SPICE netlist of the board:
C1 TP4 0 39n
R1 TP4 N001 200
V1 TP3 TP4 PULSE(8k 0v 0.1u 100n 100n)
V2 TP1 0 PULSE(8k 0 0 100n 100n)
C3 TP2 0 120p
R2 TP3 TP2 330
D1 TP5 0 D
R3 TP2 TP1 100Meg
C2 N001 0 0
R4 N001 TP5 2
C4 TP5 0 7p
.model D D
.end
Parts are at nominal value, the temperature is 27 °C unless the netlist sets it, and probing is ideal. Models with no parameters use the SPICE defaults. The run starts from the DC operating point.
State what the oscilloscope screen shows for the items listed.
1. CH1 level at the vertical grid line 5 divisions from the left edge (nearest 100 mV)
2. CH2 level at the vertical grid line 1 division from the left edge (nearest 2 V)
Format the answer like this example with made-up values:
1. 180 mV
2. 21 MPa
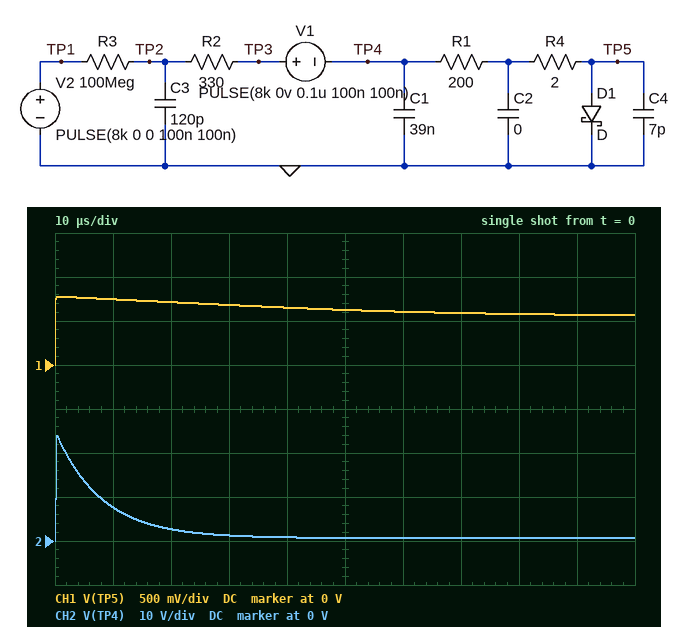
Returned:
1. 600 mV
2. 8 V
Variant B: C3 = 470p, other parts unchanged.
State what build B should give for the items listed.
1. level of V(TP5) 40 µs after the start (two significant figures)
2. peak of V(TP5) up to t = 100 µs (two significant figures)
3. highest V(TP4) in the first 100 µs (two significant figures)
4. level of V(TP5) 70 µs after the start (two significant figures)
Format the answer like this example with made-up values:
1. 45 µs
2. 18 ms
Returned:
1. 690 mV
2. 810 mV
3. 88 V
4. 610 mV
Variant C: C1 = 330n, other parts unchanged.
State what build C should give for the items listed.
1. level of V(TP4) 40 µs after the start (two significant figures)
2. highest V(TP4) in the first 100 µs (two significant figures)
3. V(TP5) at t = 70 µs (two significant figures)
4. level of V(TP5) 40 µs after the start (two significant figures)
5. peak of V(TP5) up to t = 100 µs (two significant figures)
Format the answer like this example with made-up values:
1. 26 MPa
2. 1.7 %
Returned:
1. 1.9 V
2. 2.9 V
3. 690 mV
4. 700 mV
5. 720 mV
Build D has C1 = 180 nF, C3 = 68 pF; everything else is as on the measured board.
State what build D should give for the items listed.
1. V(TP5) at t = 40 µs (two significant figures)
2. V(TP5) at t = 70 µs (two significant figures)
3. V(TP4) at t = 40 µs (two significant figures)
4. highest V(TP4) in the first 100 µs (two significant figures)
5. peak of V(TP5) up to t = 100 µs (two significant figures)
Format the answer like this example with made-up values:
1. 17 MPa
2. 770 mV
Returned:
1. 690 mV
2. 670 mV
3. 1.5 V
4. 3.0 V
5. 720 mV
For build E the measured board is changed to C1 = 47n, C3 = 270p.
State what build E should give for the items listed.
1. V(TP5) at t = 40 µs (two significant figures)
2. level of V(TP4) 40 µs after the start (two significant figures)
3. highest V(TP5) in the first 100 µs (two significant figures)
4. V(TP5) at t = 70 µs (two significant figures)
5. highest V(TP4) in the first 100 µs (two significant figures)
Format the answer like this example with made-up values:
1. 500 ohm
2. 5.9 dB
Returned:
1. 690 mV
2. 1.4 V
3. 790 mV
4. 620 mV
5. 44 V
